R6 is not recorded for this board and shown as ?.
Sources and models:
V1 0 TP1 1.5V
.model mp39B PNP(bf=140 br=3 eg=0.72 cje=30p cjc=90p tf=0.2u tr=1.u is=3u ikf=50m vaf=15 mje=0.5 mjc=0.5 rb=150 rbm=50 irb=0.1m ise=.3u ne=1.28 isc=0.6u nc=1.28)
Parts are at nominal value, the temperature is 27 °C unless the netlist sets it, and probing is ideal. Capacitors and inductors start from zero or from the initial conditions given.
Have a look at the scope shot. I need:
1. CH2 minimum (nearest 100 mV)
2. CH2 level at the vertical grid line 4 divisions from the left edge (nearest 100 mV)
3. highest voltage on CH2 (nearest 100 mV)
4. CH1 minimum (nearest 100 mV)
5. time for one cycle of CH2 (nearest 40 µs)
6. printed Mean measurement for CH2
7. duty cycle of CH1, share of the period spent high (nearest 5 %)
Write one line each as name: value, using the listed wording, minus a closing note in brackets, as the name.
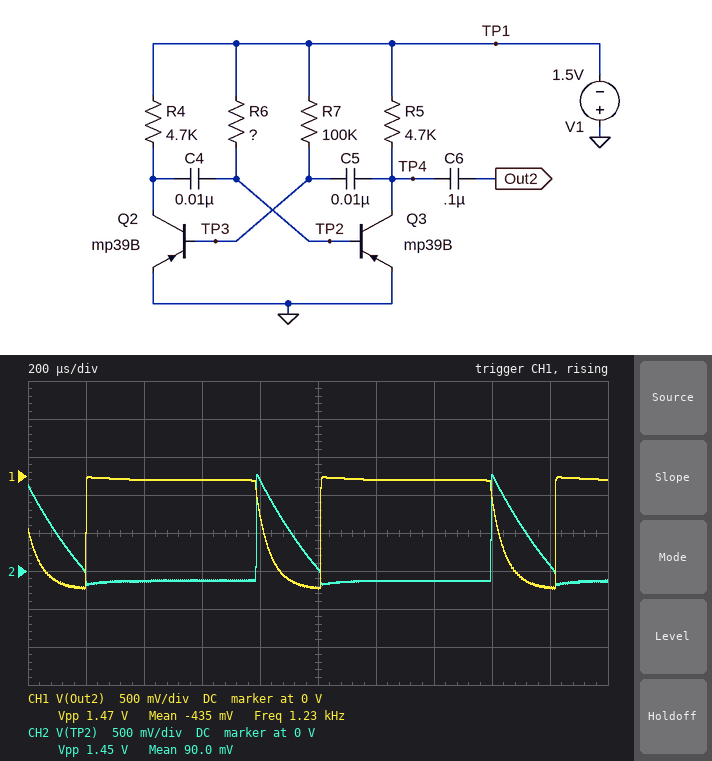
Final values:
CH2 minimum: -200 mV
CH2 level at the vertical grid line 4 divisions from the left edge: 1.2 V
highest voltage on CH2: 1.3 V
CH1 minimum: -1.5 V
time for one cycle of CH2: 800 µs
printed Mean measurement for CH2: 90.0 mV
duty cycle of CH1, share of the period spent high: 75 %
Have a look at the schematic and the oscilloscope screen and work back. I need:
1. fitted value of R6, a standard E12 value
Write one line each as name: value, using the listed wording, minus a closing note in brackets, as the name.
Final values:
fitted value of R6, a standard E12 value: 39 kΩ
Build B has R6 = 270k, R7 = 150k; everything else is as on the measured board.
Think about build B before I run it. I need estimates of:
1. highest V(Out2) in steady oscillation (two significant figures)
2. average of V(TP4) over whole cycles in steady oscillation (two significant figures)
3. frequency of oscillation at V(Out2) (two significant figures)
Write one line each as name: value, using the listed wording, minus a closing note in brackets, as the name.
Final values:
highest V(Out2) in steady oscillation: -23 mV
average of V(TP4) over whole cycles in steady oscillation: -1.2 V
frequency of oscillation at V(Out2): 740 Hz
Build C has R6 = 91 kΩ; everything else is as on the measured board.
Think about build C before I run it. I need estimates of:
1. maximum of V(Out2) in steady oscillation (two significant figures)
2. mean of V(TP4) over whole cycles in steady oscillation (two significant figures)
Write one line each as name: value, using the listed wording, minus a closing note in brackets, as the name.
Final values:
maximum of V(Out2) in steady oscillation: -20 mV
mean of V(TP4) over whole cycles in steady oscillation: -690 mV
